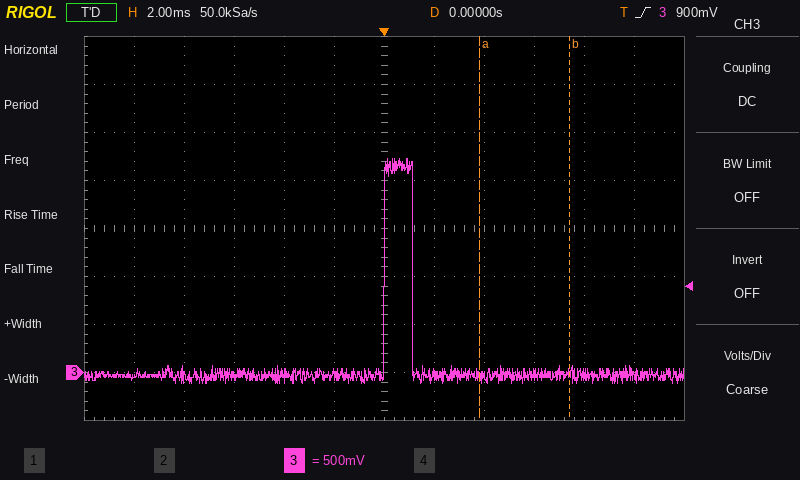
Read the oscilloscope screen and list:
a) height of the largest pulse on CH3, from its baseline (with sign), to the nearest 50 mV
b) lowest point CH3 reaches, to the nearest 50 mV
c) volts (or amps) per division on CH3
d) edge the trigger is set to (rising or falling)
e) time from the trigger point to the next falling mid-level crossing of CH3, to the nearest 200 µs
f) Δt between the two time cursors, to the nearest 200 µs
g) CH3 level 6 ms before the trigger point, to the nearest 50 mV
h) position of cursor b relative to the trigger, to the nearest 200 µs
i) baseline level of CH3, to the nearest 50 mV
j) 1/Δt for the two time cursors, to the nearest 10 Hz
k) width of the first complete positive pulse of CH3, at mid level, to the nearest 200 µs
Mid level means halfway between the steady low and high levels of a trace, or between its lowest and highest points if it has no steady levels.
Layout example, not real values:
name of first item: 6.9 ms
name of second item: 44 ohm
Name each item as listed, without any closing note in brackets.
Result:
height of the largest pulse on CH3, from its baseline (with sign), to the nearest 50 mV: +2.25 V
lowest point CH3 reaches, to the nearest 50 mV: -100 mV
volts (or amps) per division on CH3: 500 mV
edge the trigger is set to: rising
time from the trigger point to the next falling mid-level crossing of CH3, to the nearest 200 µs: 1.2 ms
Δt between the two time cursors, to the nearest 200 µs: 3.6 ms
CH3 level 6 ms before the trigger point, to the nearest 50 mV: -50 mV
position of cursor b relative to the trigger, to the nearest 200 µs: +7.4 ms
baseline level of CH3, to the nearest 50 mV: -50 mV
1/Δt for the two time cursors, to the nearest 10 Hz: 280 Hz
width of the first complete positive pulse of CH3, at mid level, to the nearest 200 µs: 1.2 ms
